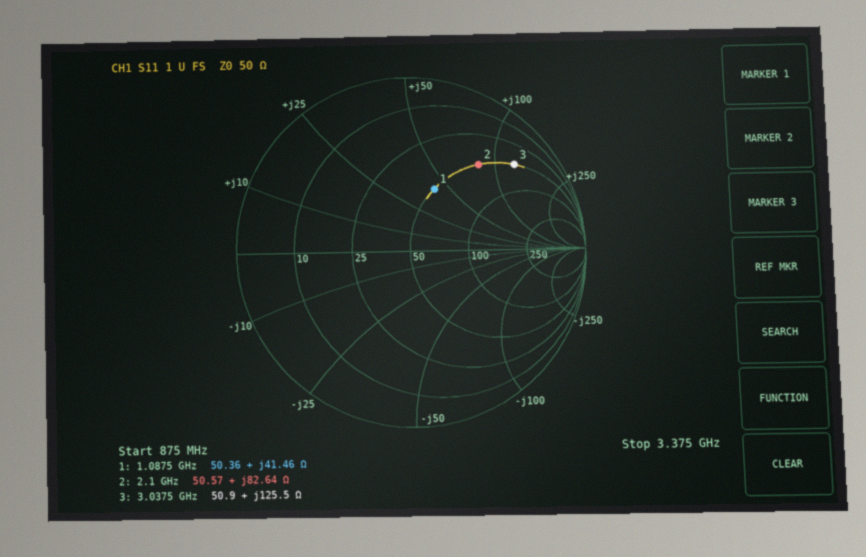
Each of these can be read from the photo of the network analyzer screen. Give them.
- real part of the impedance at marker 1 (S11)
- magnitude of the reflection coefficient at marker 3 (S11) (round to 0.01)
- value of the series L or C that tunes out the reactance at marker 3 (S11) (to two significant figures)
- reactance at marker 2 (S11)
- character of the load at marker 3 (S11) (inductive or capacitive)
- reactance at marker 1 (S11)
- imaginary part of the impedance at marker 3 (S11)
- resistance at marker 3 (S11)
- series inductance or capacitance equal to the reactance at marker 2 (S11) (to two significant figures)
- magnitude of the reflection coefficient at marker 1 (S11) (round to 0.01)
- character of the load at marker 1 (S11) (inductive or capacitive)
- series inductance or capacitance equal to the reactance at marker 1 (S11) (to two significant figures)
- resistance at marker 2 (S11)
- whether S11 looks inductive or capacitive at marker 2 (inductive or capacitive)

50.36 Ω
0.78
420 fF
+82.64 Ω
inductive
+41.46 Ω
+125.5 Ω
50.9 Ω
6.3 nH
0.38
inductive
6.1 nH
50.57 Ω
inductive
